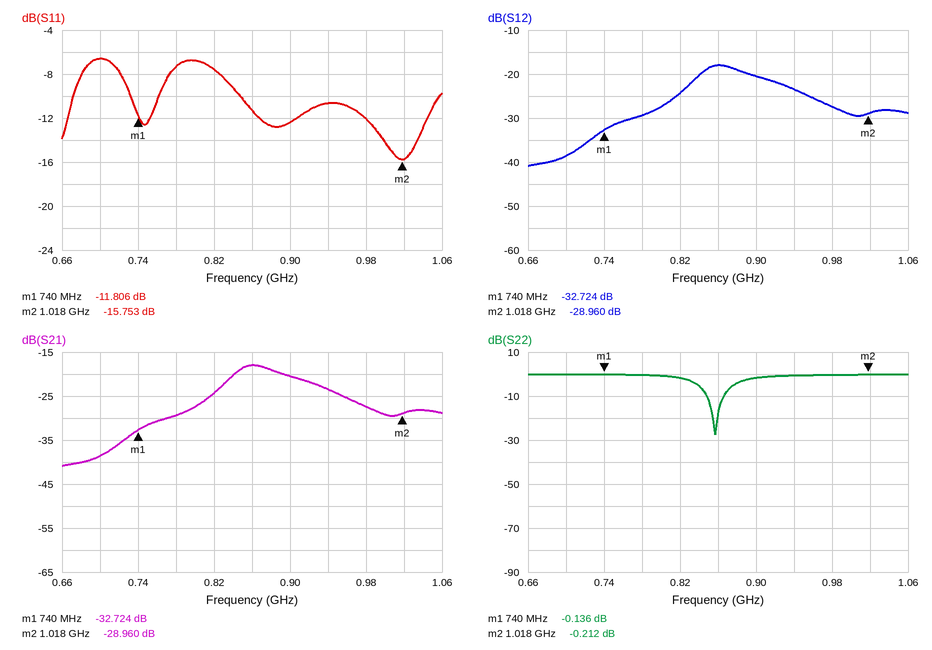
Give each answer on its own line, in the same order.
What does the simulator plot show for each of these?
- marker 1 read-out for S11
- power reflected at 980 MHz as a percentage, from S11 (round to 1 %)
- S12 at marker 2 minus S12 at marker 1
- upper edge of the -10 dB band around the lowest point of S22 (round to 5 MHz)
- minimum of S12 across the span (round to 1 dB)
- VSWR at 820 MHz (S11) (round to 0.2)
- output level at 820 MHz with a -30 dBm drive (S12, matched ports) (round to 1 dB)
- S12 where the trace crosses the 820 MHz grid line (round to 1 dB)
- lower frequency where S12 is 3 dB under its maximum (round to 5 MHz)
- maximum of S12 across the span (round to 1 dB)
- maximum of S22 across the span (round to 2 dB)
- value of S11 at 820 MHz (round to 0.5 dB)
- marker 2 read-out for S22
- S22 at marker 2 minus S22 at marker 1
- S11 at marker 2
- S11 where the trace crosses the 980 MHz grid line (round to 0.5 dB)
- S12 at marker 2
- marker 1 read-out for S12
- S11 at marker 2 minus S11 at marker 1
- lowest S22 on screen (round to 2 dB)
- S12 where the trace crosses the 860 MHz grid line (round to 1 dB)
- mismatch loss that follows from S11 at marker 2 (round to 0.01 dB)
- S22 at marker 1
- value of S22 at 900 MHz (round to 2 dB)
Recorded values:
-11.806 dB
6 %
3.764 dB
865 MHz
-41 dB
2.4
-54 dBm
-24 dB
835 MHz
-18 dB
0 dB
-7.5 dB
-0.212 dB
-0.076 dB
-15.753 dB
-12.0 dB
-28.960 dB
-32.724 dB
-3.947 dB
-28 dB
-18 dB
0.12 dB
-0.136 dB
-2 dB
